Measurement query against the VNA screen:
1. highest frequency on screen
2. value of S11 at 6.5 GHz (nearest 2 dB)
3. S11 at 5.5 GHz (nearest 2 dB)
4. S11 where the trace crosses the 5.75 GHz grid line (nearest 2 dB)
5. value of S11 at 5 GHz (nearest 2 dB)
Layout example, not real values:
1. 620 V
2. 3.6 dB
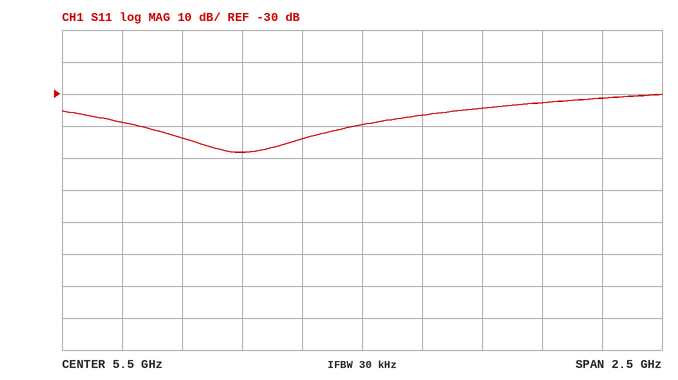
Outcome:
1. 6.75 GHz
2. -32 dB
3. -40 dB
4. -36 dB
5. -48 dB
